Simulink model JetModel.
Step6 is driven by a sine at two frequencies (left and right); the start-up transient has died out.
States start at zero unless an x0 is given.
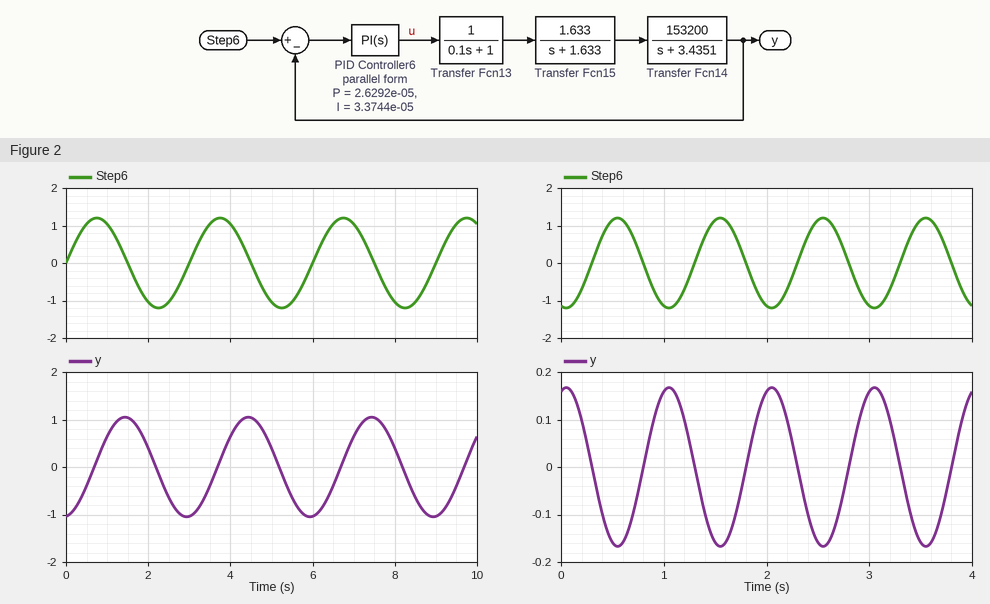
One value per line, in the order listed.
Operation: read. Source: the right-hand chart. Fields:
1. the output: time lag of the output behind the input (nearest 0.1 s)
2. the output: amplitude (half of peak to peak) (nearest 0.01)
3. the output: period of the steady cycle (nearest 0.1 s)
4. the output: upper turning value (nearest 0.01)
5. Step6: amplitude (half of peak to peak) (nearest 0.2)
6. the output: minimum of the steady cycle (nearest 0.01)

0.5 s
0.17
1.0 s
0.17
1.2
-0.17
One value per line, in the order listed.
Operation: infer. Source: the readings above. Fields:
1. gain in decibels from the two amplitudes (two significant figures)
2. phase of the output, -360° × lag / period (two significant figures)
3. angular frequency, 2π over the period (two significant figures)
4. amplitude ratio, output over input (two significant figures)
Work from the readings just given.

-17 dB
-180°
6.3 rad/s
0.14
